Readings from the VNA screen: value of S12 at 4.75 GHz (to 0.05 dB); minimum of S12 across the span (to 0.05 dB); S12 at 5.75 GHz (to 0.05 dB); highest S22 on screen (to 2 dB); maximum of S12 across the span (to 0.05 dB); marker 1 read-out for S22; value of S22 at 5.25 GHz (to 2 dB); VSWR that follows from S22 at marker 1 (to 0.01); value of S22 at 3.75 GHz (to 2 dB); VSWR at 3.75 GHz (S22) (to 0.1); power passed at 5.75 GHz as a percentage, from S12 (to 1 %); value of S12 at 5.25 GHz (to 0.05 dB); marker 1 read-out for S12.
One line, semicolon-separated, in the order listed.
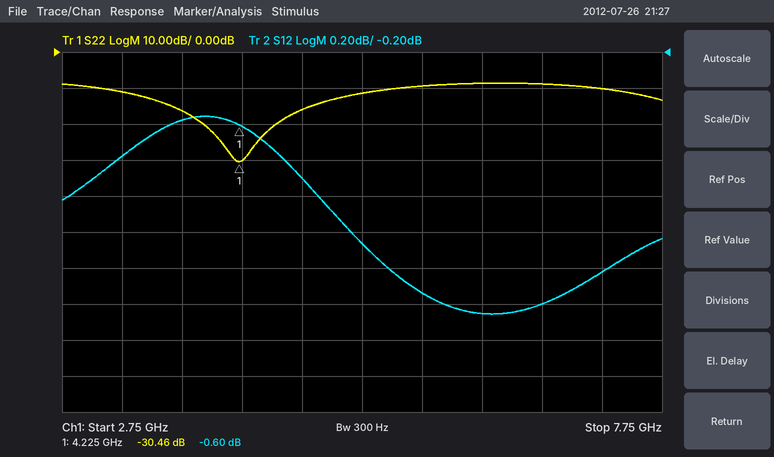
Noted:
-0.90 dB; -1.65 dB; -1.55 dB; -8 dB; -0.55 dB; -30.46 dB; -12 dB; 1.06; -16 dB; 1.4; 70 %; -1.25 dB; -0.60 dB
